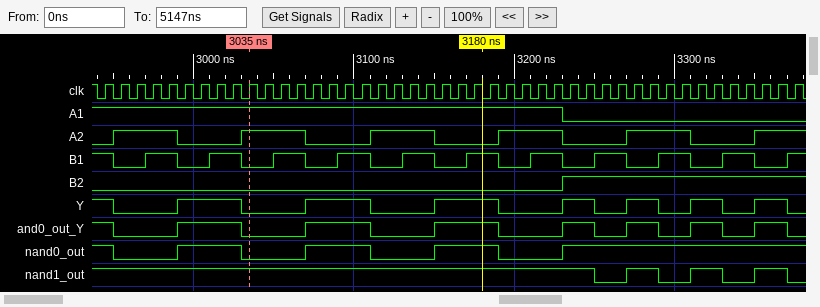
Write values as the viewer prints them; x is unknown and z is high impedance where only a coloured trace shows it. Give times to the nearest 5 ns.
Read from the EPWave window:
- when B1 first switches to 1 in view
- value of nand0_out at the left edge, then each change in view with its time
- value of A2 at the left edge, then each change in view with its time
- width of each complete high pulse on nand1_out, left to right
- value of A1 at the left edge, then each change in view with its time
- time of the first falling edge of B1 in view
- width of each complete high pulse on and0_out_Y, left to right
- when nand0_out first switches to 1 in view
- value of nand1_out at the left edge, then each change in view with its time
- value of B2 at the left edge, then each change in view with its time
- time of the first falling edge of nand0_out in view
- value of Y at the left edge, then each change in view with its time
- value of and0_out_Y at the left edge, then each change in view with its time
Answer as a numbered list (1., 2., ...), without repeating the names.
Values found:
1. 2970 ns
2. 1, 0 at 2950 ns, 1 at 2990 ns, 0 at 3030 ns, 1 at 3070 ns, 0 at 3110 ns, 1 at 3150 ns, 0 at 3190 ns, 1 at 3230 ns
3. 0, 1 at 2950 ns, 0 at 2990 ns, 1 at 3030 ns, 0 at 3070 ns, 1 at 3110 ns, 0 at 3150 ns, 1 at 3190 ns, 0 at 3230 ns, 1 at 3270 ns, 0 at 3310 ns, 1 at 3350 ns
4. 20 ns, 20 ns, 20 ns
5. 1, 0 at 3230 ns
6. 2950 ns
7. 40 ns, 40 ns, 40 ns, 20 ns, 20 ns, 20 ns, 20 ns
8. 2990 ns
9. 1, 0 at 3250 ns, 1 at 3270 ns, 0 at 3290 ns, 1 at 3310 ns, 0 at 3330 ns, 1 at 3350 ns, 0 at 3370 ns
10. 0, 1 at 3230 ns
11. 2950 ns
12. 1, 0 at 2950 ns, 1 at 2990 ns, 0 at 3030 ns, 1 at 3070 ns, 0 at 3110 ns, 1 at 3150 ns, 0 at 3190 ns, 1 at 3230 ns, 0 at 3250 ns, 1 at 3270 ns, 0 at 3290 ns, 1 at 3310 ns, 0 at 3330 ns, 1 at 3350 ns, 0 at 3370 ns
13. 1, 0 at 2950 ns, 1 at 2990 ns, 0 at 3030 ns, 1 at 3070 ns, 0 at 3110 ns, 1 at 3150 ns, 0 at 3190 ns, 1 at 3230 ns, 0 at 3250 ns, 1 at 3270 ns, 0 at 3290 ns, 1 at 3310 ns, 0 at 3330 ns, 1 at 3350 ns, 0 at 3370 ns
